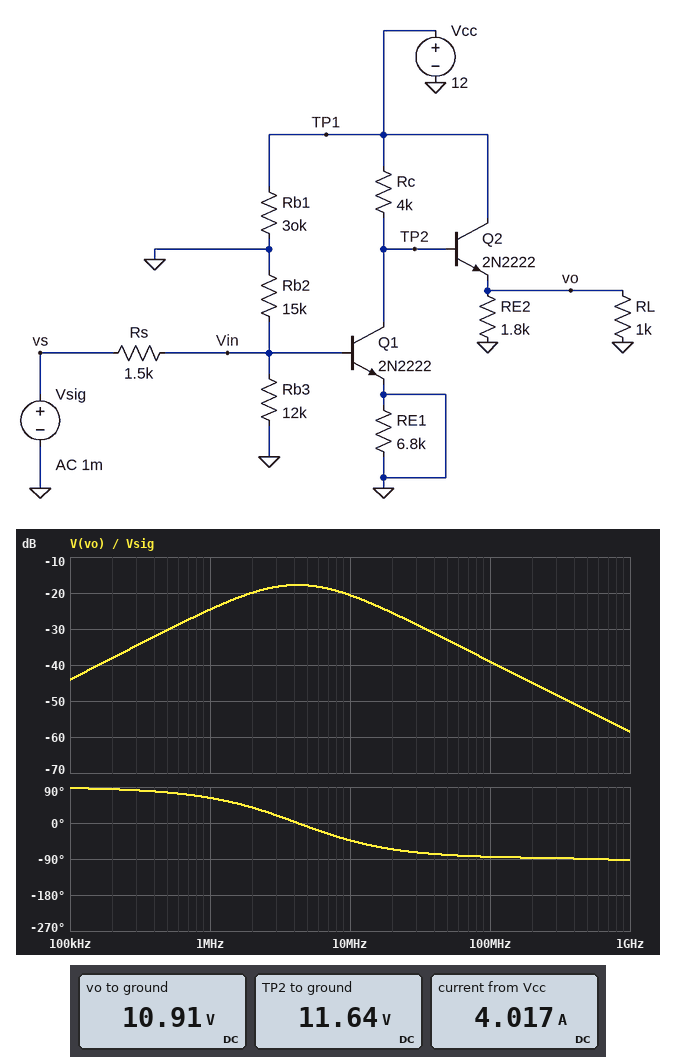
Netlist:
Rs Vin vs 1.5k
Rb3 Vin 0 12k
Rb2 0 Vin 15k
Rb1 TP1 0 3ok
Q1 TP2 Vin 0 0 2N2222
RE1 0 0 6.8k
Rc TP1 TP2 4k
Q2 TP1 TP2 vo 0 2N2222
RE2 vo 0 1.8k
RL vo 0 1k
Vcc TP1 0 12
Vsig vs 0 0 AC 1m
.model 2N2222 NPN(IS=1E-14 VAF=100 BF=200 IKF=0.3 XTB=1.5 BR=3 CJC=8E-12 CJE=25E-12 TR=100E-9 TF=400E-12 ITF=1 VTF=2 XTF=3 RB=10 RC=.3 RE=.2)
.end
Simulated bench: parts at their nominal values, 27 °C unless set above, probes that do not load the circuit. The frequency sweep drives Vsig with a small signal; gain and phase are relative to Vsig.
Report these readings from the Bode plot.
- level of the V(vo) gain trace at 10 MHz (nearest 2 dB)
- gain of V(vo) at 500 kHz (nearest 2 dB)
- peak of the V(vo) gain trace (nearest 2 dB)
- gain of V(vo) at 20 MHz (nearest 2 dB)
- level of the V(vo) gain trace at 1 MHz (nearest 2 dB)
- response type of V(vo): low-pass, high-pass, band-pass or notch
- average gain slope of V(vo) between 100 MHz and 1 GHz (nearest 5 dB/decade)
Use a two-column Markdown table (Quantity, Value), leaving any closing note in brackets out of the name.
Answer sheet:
| Quantity | Value |
|---|---|
| level of the V(vo) gain trace at 10 MHz | -20 dB |
| gain of V(vo) at 500 kHz | -30 dB |
| peak of the V(vo) gain trace | -18 dB |
| gain of V(vo) at 20 MHz | -26 dB |
| level of the V(vo) gain trace at 1 MHz | -24 dB |
| response type of V(vo): low-pass, high-pass, band-pass or notch | band-pass |
| average gain slope of V(vo) between 100 MHz and 1 GHz | -20 dB/decade |
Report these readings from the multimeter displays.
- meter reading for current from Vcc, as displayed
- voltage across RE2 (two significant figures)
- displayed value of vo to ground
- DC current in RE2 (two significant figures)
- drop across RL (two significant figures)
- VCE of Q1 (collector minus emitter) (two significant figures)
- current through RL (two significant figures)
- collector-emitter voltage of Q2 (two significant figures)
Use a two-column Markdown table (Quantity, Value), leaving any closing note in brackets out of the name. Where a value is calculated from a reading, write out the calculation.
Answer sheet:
| Quantity | Value |
|---|---|
| meter reading for current from Vcc, as displayed | 4.017 A |
| voltage across RE2 | 10.91 V = 11 V |
| displayed value of vo to ground | 10.91 V |
| DC current in RE2 | (10.91 V) / 1.8 kΩ = 6.1 mA |
| drop across RL | 10.91 V = 11 V |
| VCE of Q1 (collector minus emitter) | 11.64 V = 12 V |
| current through RL | (10.91 V) / 1 kΩ = 11 mA |
| collector-emitter voltage of Q2 | 12 V - 10.91 V = 1.1 V |
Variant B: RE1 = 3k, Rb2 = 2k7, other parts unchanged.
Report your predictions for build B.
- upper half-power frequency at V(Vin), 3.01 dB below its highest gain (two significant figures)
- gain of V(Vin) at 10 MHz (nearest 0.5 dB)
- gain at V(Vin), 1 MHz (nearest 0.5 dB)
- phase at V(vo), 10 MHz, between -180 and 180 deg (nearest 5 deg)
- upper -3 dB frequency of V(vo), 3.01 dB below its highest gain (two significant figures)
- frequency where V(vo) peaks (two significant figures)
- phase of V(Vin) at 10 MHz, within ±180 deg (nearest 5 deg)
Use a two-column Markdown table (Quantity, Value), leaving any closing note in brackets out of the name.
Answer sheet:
| Quantity | Value |
|---|---|
| upper half-power frequency at V(Vin), 3.01 dB below its highest gain | 6.3 MHz |
| gain of V(Vin) at 10 MHz | -10.0 dB |
| gain at V(Vin), 1 MHz | -4.5 dB |
| phase at V(vo), 10 MHz, between -180 and 180 deg | -35 deg |
| upper -3 dB frequency of V(vo), 3.01 dB below its highest gain | 12 MHz |
| frequency where V(vo) peaks | 4.9 MHz |
| phase of V(Vin) at 10 MHz, within ±180 deg | -55 deg |
